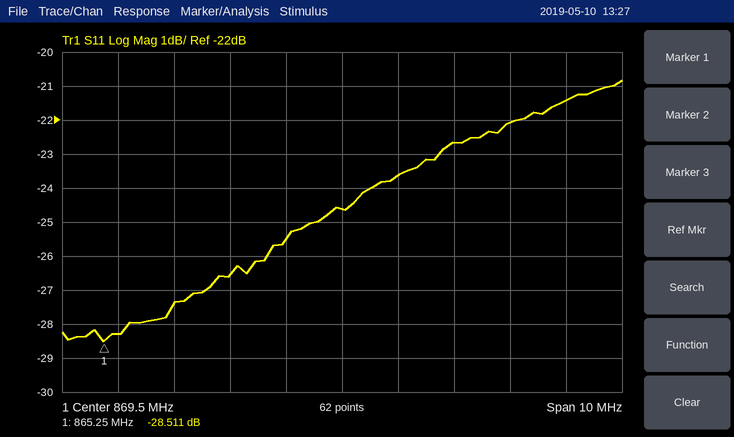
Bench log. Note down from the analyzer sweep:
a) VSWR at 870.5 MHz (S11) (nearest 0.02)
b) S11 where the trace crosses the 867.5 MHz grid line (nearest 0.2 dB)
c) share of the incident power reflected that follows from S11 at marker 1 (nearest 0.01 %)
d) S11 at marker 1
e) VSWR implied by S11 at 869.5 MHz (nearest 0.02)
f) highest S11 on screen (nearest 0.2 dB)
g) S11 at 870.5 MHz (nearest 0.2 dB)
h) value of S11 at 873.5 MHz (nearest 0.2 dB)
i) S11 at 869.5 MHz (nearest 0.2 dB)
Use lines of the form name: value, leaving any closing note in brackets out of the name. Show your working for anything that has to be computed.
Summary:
VSWR at 870.5 MHz (S11): |Γ| = 10^(-23.6/20) = 0.0661; VSWR = (1 + 0.0661)/(1 − 0.0661) ≈ 1.14
S11 where the trace crosses the 867.5 MHz grid line: -26.6 dB
share of the incident power reflected that follows from S11 at marker 1: 10^(-28.511/10) ≈ 0.14 %
S11 at marker 1: -28.511 dB
VSWR implied by S11 at 869.5 MHz: |Γ| = 10^(-24.6/20) = 0.0589; VSWR = (1 + 0.0589)/(1 − 0.0589) ≈ 1.13, so 1.12 to the nearest 0.02
highest S11 on screen: -20.8 dB
S11 at 870.5 MHz: -23.6 dB
value of S11 at 873.5 MHz: -21.4 dB
S11 at 869.5 MHz: -24.6 dB
